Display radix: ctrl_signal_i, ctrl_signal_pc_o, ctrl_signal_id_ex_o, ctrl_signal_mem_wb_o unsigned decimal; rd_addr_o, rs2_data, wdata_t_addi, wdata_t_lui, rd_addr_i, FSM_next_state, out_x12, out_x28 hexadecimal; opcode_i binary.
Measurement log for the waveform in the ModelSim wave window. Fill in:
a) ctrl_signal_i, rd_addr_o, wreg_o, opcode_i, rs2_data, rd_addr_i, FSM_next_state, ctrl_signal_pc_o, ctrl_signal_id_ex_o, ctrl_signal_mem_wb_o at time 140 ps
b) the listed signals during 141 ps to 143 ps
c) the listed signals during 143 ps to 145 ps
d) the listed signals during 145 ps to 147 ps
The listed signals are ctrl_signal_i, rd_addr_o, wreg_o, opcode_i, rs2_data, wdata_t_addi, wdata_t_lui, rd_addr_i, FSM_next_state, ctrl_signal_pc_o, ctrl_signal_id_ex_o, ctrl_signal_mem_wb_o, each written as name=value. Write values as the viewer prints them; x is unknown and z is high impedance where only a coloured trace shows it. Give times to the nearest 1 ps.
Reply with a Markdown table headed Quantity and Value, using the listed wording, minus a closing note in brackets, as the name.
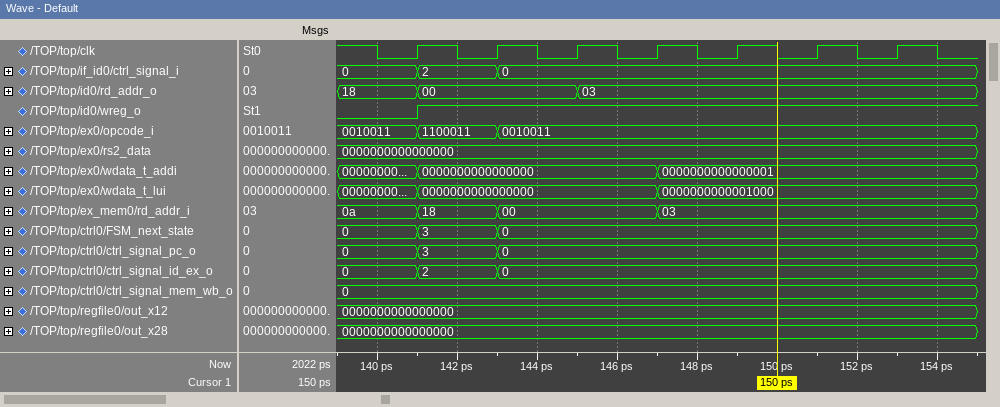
| Quantity | Value |
|---|---|
| ctrl_signal_i, rd_addr_o, wreg_o, opcode_i, rs2_data, rd_addr_i, FSM_next_state, ctrl_signal_pc_o, ctrl_signal_id_ex_o, ctrl_signal_mem_wb_o at time 140 ps | ctrl_signal_i=0, rd_addr_o=18, wreg_o=0, opcode_i=0010011, rs2_data=0000000000000000, rd_addr_i=0a, FSM_next_state=0, ctrl_signal_pc_o=0, ctrl_signal_id_ex_o=0, ctrl_signal_mem_wb_o=0 |
| the listed signals during 141 ps to 143 ps | ctrl_signal_i=2, rd_addr_o=00, wreg_o=1, opcode_i=1100011, rs2_data=0000000000000000, wdata_t_addi=0000000000000000, wdata_t_lui=0000000000000000, rd_addr_i=18, FSM_next_state=3, ctrl_signal_pc_o=3, ctrl_signal_id_ex_o=2, ctrl_signal_mem_wb_o=0 |
| the listed signals during 143 ps to 145 ps | ctrl_signal_i=0, rd_addr_o=00, wreg_o=1, opcode_i=0010011, rs2_data=0000000000000000, wdata_t_addi=0000000000000000, wdata_t_lui=0000000000000000, rd_addr_i=00, FSM_next_state=0, ctrl_signal_pc_o=0, ctrl_signal_id_ex_o=0, ctrl_signal_mem_wb_o=0 |
| the listed signals during 145 ps to 147 ps | ctrl_signal_i=0, rd_addr_o=03, wreg_o=1, opcode_i=0010011, rs2_data=0000000000000000, wdata_t_addi=0000000000000000, wdata_t_lui=0000000000000000, rd_addr_i=00, FSM_next_state=0, ctrl_signal_pc_o=0, ctrl_signal_id_ex_o=0, ctrl_signal_mem_wb_o=0 |
